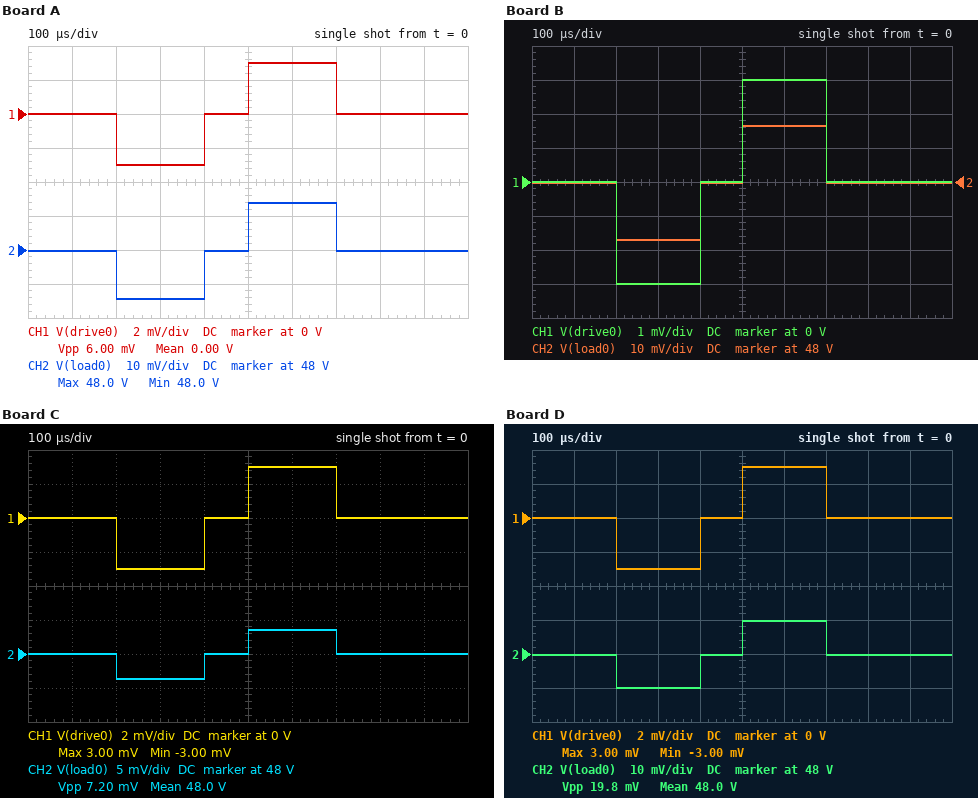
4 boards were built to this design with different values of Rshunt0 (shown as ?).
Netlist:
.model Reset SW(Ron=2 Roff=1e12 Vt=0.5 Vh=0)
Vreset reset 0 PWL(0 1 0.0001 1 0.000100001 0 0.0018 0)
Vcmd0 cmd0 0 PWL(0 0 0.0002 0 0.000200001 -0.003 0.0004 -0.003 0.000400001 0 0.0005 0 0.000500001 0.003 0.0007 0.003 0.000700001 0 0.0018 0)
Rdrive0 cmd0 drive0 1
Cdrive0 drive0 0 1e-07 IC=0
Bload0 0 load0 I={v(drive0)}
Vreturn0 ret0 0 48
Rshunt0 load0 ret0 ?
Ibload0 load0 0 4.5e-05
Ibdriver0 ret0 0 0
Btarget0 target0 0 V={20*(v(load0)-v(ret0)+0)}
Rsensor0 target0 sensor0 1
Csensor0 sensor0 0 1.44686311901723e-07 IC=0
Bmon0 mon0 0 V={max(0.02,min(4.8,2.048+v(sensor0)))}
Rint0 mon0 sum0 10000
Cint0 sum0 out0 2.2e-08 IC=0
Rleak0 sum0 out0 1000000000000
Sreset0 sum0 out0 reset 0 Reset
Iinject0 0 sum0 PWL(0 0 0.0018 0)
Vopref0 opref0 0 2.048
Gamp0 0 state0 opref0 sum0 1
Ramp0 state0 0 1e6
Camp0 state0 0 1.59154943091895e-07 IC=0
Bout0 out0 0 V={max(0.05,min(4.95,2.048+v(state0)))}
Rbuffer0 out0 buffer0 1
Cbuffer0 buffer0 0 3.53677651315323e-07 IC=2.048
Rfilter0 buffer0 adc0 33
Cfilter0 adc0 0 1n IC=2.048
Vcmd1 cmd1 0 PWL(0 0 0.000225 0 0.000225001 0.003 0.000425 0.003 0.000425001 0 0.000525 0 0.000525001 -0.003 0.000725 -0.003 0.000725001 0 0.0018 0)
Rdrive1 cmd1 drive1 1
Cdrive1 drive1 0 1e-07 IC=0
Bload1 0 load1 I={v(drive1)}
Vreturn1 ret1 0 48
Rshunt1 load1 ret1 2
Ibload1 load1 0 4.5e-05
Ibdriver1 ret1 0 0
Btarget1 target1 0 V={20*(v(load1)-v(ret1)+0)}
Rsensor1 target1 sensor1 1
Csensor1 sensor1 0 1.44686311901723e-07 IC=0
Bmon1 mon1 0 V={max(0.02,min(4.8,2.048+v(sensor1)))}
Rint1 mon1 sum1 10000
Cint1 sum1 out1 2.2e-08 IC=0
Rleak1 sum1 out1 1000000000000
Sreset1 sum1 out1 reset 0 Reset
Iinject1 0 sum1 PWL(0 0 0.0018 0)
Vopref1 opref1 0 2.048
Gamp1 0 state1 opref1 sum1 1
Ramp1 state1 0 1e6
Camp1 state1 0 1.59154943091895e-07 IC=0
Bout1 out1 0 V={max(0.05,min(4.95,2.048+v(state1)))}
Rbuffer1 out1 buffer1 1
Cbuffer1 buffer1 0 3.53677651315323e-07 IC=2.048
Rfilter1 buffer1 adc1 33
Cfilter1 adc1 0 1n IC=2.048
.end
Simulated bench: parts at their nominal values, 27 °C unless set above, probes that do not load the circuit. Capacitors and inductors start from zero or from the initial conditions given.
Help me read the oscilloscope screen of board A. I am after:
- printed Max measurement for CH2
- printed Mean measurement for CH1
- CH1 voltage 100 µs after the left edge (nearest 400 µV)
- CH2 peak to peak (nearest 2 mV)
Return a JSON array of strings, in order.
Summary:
["48.0 V", "0.00 V", "0 V", "28 mV"]
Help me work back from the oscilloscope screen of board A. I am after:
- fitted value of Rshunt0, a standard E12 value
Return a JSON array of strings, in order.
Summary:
["4.7 Ω"]
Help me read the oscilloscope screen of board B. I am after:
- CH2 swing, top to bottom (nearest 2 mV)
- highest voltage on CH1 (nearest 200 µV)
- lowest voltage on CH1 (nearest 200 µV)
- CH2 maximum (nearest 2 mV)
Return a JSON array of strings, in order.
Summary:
["34 mV", "3.0 mV", "-3.0 mV", "48.016 V"]
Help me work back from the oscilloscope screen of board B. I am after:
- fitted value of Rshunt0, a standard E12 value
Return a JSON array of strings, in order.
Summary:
["5.6 Ω"]
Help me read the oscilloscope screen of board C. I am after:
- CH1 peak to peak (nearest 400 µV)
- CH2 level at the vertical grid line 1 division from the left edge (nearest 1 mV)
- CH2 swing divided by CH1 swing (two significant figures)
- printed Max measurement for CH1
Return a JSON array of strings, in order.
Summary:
["6.0 mV", "48.000 V", "1.2", "3.00 mV"]
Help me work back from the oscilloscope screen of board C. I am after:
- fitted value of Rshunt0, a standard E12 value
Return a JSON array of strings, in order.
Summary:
["1.2 Ω"]
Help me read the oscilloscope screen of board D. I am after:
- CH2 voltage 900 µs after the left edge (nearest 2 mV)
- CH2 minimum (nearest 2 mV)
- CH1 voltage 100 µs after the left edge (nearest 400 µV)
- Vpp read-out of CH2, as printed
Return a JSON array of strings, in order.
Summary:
["48.000 V", "47.990 V", "0 V", "19.8 mV"]
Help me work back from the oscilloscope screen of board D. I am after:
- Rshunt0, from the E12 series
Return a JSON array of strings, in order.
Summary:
["3.3 Ω"]
